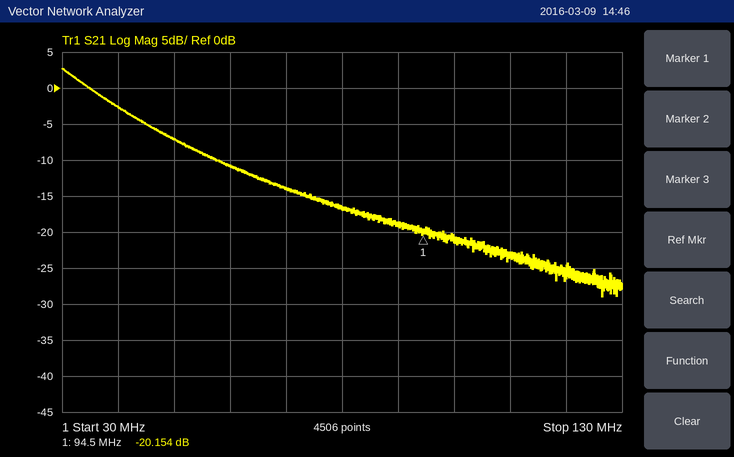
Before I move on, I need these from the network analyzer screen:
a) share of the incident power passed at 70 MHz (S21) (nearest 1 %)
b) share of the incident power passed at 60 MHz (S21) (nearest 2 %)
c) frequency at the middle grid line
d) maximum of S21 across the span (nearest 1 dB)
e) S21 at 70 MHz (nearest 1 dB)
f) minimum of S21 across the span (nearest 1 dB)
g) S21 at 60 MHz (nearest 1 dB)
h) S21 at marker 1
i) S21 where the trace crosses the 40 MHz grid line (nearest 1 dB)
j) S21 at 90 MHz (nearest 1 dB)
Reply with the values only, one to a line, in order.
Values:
4 %
8 %
80 MHz
3 dB
-14 dB
-29 dB
-11 dB
-20.154 dB
-3 dB
-19 dB
